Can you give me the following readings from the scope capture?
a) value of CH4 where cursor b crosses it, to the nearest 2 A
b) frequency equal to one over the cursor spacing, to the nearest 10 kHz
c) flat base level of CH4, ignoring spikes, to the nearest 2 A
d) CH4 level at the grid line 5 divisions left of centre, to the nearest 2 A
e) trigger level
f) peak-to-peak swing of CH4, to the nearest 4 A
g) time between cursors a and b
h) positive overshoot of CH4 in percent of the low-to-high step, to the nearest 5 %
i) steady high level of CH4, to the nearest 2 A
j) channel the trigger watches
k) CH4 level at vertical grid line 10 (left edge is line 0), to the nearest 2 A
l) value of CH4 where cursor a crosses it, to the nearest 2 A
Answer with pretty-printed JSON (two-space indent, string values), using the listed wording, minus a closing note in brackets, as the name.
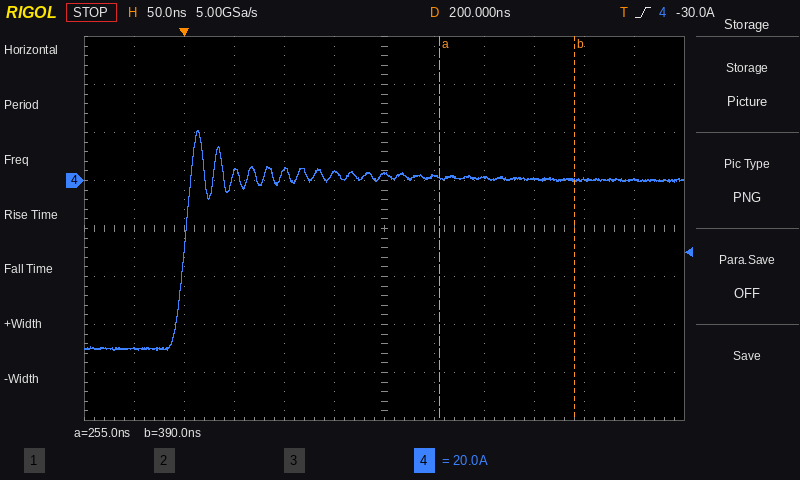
{
  "value of CH4 where cursor b crosses it, to the nearest 2 A": "0 A",
  "frequency equal to one over the cursor spacing, to the nearest 10 kHz": "7.41 MHz",
  "flat base level of CH4, ignoring spikes, to the nearest 2 A": "-70 A",
  "CH4 level at the grid line 5 divisions left of centre, to the nearest 2 A": "-70 A",
  "trigger level": "-30.0 A",
  "peak-to-peak swing of CH4, to the nearest 4 A": "92 A",
  "time between cursors a and b": "135 ns",
  "positive overshoot of CH4 in percent of the low-to-high step, to the nearest 5 %": "30 %",
  "steady high level of CH4, to the nearest 2 A": "0 A",
  "channel the trigger watches": "CH4",
  "CH4 level at vertical grid line 10 (left edge is line 0), to the nearest 2 A": "0 A",
  "value of CH4 where cursor a crosses it, to the nearest 2 A": "2 A"
}
